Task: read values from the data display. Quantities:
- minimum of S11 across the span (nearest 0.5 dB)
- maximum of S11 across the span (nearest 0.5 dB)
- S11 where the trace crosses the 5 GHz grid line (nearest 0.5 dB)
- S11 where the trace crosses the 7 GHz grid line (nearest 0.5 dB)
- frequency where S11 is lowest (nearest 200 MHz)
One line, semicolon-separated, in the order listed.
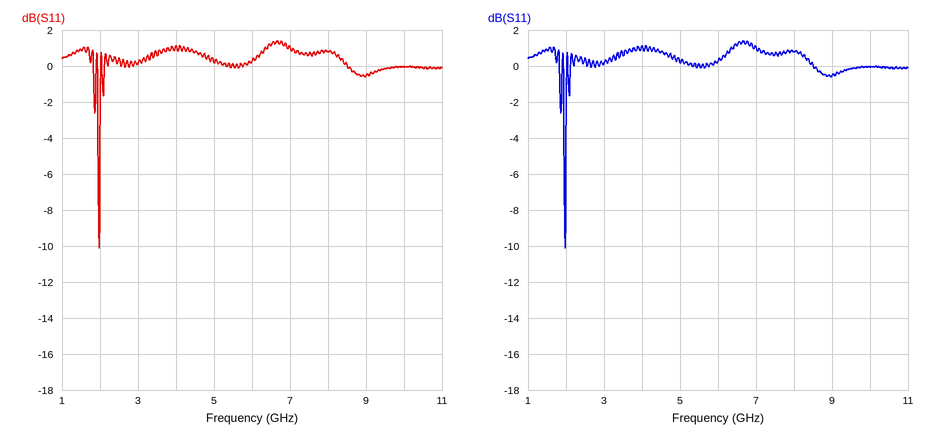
-10.0 dB; 1.5 dB; 0.0 dB; 1.0 dB; 2.0 GHz
